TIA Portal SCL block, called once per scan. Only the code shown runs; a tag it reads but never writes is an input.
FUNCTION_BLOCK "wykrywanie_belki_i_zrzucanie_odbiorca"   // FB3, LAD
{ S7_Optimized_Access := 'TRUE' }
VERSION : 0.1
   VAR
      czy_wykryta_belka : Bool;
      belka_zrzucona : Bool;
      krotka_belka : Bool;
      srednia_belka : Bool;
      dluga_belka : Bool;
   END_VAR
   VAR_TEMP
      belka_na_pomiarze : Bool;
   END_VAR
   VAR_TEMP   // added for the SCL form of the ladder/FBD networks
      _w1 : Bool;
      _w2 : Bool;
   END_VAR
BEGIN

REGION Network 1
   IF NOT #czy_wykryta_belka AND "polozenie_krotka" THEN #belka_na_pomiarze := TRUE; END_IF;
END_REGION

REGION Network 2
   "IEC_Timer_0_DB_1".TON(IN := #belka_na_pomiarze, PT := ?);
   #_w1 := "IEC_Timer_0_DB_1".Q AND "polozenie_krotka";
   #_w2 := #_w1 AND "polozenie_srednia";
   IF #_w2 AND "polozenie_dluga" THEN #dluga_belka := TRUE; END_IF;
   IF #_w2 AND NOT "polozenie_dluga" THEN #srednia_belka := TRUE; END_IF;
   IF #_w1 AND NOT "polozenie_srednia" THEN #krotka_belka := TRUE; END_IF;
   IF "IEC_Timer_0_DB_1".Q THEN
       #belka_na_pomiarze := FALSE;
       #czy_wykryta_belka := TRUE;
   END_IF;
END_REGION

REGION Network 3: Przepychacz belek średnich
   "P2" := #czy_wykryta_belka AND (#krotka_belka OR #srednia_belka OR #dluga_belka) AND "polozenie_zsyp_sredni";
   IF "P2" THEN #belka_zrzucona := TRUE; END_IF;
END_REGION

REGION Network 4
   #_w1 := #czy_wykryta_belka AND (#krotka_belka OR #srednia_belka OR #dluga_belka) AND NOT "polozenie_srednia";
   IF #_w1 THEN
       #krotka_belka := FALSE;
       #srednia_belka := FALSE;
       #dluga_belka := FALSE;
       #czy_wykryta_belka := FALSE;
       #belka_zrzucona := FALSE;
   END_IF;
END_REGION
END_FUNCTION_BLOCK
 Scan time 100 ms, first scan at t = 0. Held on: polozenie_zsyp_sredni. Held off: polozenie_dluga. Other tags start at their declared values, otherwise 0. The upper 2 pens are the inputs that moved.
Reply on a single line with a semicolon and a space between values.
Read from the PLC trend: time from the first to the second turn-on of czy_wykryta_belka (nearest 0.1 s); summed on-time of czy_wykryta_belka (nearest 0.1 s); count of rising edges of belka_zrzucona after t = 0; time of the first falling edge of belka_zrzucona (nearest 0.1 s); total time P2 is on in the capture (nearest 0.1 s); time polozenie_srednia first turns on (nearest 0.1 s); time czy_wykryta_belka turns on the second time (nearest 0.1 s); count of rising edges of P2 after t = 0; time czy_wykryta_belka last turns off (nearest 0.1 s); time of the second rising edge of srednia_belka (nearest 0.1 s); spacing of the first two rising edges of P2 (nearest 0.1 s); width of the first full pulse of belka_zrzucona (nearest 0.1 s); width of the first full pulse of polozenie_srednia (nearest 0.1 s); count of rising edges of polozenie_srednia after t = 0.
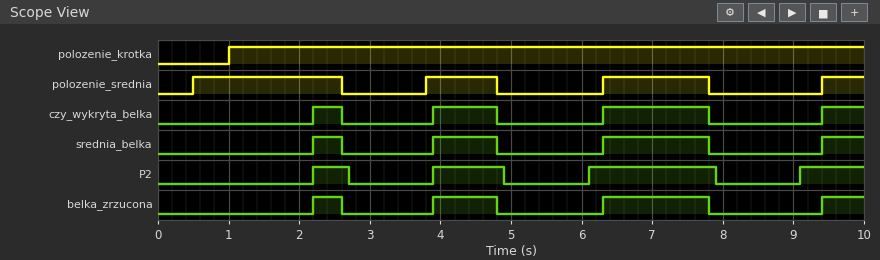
1.7 s; 3.4 s; 4; 2.6 s; 4.2 s; 0.5 s; 3.9 s; 4; 7.8 s; 3.9 s; 1.7 s; 0.4 s; 2.1 s; 4
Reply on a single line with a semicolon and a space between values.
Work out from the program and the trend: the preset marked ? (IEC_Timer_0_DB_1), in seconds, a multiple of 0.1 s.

1.2 s
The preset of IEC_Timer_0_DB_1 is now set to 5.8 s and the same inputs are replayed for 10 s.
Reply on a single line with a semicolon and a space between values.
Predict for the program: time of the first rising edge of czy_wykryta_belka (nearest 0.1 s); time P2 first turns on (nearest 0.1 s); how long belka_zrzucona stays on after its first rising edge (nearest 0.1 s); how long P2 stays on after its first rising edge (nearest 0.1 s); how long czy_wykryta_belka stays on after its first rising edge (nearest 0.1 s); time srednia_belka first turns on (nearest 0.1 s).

6.8 s; 6.8 s; 1.0 s; 1.1 s; 1.0 s; 6.8 s
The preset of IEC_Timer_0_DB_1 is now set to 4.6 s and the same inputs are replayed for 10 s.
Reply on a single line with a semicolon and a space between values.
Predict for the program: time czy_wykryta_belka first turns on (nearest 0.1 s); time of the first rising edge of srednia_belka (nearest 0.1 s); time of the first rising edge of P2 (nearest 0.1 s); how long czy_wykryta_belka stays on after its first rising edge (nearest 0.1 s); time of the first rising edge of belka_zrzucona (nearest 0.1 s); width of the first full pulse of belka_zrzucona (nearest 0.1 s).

6.3 s; 6.3 s; 5.6 s; 1.5 s; 6.3 s; 1.5 s
